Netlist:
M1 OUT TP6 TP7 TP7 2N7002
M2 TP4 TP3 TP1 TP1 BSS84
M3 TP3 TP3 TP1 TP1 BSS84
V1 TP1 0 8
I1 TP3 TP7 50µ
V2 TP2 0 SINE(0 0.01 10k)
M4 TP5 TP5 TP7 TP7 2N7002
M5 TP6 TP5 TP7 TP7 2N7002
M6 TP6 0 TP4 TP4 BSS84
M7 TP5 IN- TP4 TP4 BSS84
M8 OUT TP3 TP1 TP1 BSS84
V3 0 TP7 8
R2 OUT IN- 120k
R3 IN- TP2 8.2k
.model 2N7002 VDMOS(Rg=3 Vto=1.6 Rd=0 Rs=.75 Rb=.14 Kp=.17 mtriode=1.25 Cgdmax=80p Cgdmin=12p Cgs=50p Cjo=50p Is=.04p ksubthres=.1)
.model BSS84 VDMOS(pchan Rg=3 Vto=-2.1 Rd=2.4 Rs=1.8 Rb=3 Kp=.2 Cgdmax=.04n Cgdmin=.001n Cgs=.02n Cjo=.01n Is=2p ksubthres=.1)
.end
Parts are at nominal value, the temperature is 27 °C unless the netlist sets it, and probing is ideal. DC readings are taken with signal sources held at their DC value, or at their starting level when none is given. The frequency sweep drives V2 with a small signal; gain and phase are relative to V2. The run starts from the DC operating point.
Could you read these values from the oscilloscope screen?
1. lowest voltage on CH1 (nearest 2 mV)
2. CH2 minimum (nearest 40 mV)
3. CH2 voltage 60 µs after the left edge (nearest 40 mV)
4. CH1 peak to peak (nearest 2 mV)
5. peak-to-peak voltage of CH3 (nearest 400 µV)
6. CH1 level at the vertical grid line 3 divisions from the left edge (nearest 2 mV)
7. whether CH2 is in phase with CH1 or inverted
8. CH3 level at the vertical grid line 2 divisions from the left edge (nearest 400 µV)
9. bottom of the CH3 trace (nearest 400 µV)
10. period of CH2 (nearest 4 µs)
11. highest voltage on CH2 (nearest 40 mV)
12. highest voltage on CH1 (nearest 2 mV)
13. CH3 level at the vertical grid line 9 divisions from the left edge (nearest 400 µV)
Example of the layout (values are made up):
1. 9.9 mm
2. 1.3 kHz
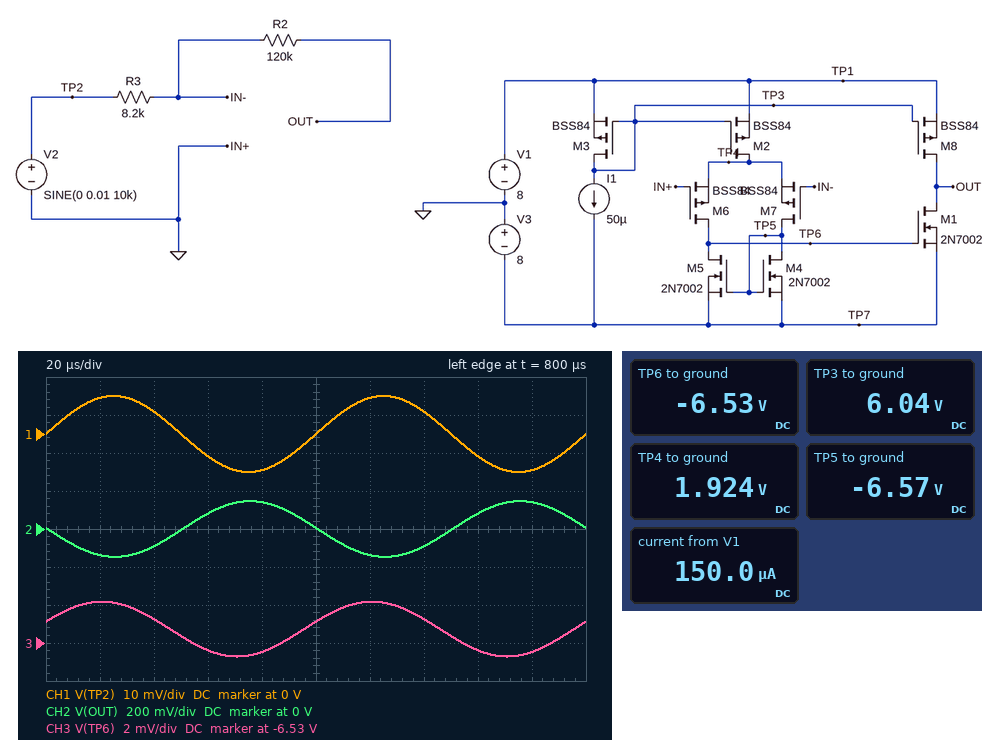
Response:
1. -10 mV
2. -160 mV
3. 80 mV
4. 20 mV
5. 2.8 mV
6. -6 mV
7. inverted
8. -6.5288 V
9. -6.5308 V
10. 100 µs
11. 160 mV
12. 10 mV
13. -6.5304 V
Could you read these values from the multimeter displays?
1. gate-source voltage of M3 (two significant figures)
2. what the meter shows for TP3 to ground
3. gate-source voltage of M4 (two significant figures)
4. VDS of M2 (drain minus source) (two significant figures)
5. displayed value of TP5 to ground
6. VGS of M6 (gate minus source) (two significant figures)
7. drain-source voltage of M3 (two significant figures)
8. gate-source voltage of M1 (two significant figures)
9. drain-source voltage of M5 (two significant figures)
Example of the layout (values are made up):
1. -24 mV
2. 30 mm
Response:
1. -2.0 V
2. 6.04 V
3. 1.4 V
4. -6.1 V
5. -6.57 V
6. -1.9 V
7. -2.0 V
8. 1.5 V
9. 1.5 V
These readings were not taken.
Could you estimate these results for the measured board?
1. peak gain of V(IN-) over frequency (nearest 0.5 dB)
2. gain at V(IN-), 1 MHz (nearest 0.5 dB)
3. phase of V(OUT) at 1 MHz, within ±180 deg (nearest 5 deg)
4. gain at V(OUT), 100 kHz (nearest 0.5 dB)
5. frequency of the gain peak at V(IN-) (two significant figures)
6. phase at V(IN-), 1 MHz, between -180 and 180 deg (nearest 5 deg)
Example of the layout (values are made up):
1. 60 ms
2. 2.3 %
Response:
1. 6.0 dB
2. -2.0 dB
3. -45 deg
4. 24.5 dB
5. 260 kHz
6. -35 deg
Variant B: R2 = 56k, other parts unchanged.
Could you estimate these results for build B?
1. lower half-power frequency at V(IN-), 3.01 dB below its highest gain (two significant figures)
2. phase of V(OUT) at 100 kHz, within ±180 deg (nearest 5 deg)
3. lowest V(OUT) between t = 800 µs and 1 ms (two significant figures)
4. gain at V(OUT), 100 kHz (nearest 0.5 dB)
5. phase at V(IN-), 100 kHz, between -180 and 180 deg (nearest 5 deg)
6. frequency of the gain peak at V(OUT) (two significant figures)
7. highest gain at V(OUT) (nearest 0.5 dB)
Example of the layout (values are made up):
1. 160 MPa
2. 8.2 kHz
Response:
1. 290 kHz
2. 165 deg
3. -68 mV
4. 17.5 dB
5. 100 deg
6. 320 kHz
7. 26.0 dB
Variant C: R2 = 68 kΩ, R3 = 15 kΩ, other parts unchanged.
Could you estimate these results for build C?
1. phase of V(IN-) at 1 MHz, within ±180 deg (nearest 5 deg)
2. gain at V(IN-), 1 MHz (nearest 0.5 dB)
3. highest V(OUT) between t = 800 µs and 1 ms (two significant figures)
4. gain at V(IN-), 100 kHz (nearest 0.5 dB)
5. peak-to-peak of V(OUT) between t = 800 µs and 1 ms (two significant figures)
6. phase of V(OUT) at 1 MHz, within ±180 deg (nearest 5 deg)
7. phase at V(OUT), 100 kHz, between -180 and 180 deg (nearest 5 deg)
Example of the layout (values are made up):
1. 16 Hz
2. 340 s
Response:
1. -55 deg
2. -4.5 dB
3. 45 mV
4. -17.0 dB
5. 91 mV
6. -65 deg
7. 170 deg
